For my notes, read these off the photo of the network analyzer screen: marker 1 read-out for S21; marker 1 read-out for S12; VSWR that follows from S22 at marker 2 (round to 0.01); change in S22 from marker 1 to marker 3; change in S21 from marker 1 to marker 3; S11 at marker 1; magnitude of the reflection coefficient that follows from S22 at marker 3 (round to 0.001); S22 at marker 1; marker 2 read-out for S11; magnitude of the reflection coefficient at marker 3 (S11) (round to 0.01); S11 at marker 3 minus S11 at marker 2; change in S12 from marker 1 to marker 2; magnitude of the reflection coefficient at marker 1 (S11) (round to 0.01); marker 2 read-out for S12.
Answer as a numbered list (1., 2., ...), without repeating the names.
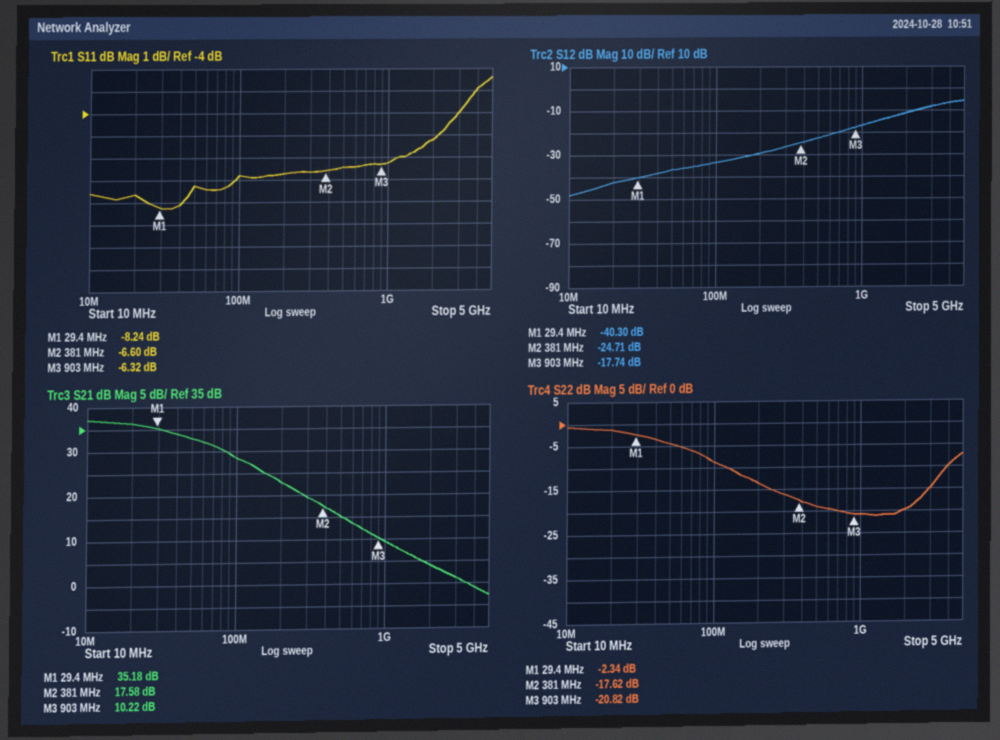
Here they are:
1. 35.18 dB
2. -40.30 dB
3. 1.30
4. -18.48 dB
5. -24.96 dB
6. -8.24 dB
7. 0.091
8. -2.34 dB
9. -6.60 dB
10. 0.48
11. 0.28 dB
12. 15.59 dB
13. 0.39
14. -24.71 dB
